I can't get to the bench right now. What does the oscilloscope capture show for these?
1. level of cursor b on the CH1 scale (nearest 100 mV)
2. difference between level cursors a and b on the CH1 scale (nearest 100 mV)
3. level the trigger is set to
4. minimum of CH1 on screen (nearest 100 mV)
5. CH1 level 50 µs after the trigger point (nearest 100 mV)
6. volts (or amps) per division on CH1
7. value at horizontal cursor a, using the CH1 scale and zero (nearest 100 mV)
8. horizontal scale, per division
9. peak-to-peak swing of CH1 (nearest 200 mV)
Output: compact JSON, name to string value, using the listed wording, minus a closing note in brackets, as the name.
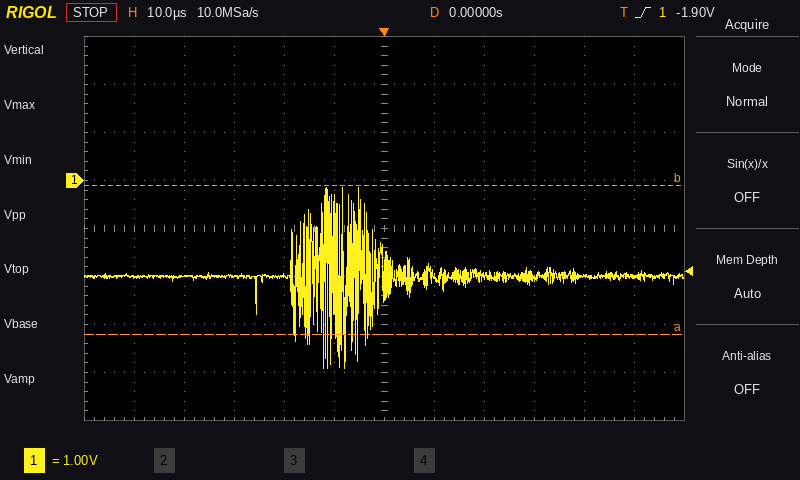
{"level of cursor b on the CH1 scale": "-100 mV", "difference between level cursors a and b on the CH1 scale": "3.1 V", "level the trigger is set to": "-1.90 V", "minimum of CH1 on screen": "-3.9 V", "CH1 level 50 µs after the trigger point": "-2.0 V", "volts (or amps) per division on CH1": "1 V", "value at horizontal cursor a, using the CH1 scale and zero": "-3.2 V", "horizontal scale, per division": "10 µs", "peak-to-peak swing of CH1": "3.8 V"}
